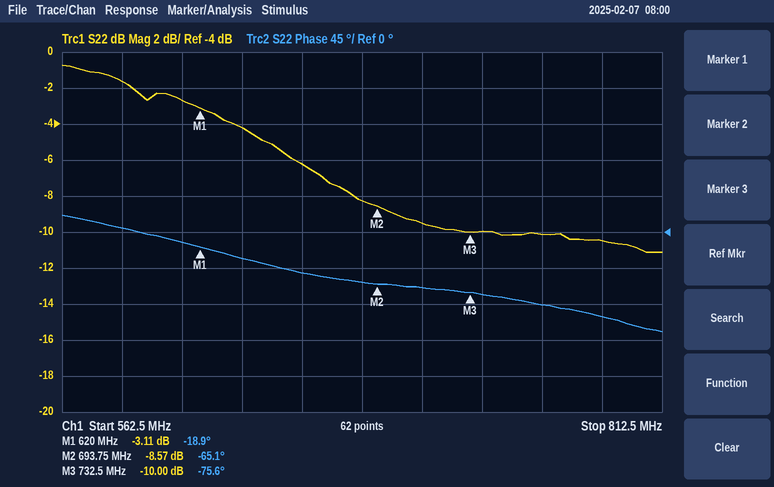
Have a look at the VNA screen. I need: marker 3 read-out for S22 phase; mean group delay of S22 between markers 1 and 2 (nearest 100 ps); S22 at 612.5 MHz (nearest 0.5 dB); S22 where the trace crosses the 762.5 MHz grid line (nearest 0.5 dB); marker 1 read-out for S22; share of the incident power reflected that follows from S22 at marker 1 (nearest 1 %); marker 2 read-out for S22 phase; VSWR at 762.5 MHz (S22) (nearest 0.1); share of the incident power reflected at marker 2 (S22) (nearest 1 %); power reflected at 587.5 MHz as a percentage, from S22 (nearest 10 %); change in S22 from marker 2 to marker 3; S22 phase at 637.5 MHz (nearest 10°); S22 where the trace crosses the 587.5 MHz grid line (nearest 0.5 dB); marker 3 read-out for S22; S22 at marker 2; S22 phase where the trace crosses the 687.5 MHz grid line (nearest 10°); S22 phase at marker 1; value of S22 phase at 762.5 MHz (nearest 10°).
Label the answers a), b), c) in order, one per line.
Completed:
a) -75.6°
b) 1.7 ns
c) -2.5 dB
d) -10.0 dB
e) -3.11 dB
f) 49 %
g) -65.1°
h) 1.9
i) 14 %
j) 70 %
k) -1.43 dB
l) -30°
m) -1.5 dB
n) -10.00 dB
o) -8.57 dB
p) -60°
q) -18.9°
r) -90°
